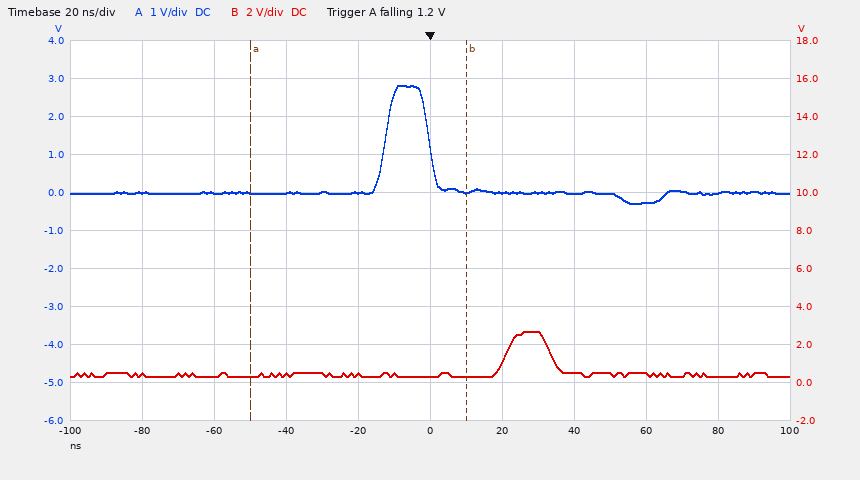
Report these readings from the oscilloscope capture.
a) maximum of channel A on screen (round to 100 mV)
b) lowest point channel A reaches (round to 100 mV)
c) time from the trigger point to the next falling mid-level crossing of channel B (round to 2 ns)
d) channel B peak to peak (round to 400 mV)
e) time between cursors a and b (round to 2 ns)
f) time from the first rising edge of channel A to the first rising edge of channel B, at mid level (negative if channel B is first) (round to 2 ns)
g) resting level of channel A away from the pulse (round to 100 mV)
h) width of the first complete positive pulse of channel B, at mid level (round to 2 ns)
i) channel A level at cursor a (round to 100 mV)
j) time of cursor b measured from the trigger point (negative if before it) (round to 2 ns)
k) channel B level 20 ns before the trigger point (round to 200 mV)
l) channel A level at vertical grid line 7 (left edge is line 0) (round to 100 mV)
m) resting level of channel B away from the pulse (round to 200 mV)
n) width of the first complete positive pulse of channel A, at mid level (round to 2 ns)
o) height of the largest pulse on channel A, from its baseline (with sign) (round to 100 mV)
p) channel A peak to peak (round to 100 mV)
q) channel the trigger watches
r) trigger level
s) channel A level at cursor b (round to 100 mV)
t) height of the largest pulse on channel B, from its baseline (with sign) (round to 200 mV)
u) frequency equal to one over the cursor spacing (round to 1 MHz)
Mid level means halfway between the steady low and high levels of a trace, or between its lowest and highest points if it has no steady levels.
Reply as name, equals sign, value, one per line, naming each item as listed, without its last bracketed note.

maximum of channel A on screen = 2.8 V
lowest point channel A reaches = -300 mV
time from the trigger point to the next falling mid-level crossing of channel B = 34 ns
channel B peak to peak = 2.4 V
time between cursors a and b = 60 ns
time from the first rising edge of channel A to the first rising edge of channel B, at mid level (negative if channel B is first) = +34 ns
resting level of channel A away from the pulse = 0.0 V
width of the first complete positive pulse of channel B, at mid level = 12 ns
channel A level at cursor a = 0.0 V
time of cursor b measured from the trigger point (negative if before it) = +10 ns
channel B level 20 ns before the trigger point = 400 mV
channel A level at vertical grid line 7 (left edge is line 0) = 0.0 V
resting level of channel B away from the pulse = 400 mV
width of the first complete positive pulse of channel A, at mid level = 12 ns
height of the largest pulse on channel A, from its baseline (with sign) = +2.8 V
channel A peak to peak = 3.1 V
channel the trigger watches = channel A
trigger level = 1.2 V
channel A level at cursor b = 0.0 V
height of the largest pulse on channel B, from its baseline (with sign) = +2.4 V
frequency equal to one over the cursor spacing = 17 MHz
